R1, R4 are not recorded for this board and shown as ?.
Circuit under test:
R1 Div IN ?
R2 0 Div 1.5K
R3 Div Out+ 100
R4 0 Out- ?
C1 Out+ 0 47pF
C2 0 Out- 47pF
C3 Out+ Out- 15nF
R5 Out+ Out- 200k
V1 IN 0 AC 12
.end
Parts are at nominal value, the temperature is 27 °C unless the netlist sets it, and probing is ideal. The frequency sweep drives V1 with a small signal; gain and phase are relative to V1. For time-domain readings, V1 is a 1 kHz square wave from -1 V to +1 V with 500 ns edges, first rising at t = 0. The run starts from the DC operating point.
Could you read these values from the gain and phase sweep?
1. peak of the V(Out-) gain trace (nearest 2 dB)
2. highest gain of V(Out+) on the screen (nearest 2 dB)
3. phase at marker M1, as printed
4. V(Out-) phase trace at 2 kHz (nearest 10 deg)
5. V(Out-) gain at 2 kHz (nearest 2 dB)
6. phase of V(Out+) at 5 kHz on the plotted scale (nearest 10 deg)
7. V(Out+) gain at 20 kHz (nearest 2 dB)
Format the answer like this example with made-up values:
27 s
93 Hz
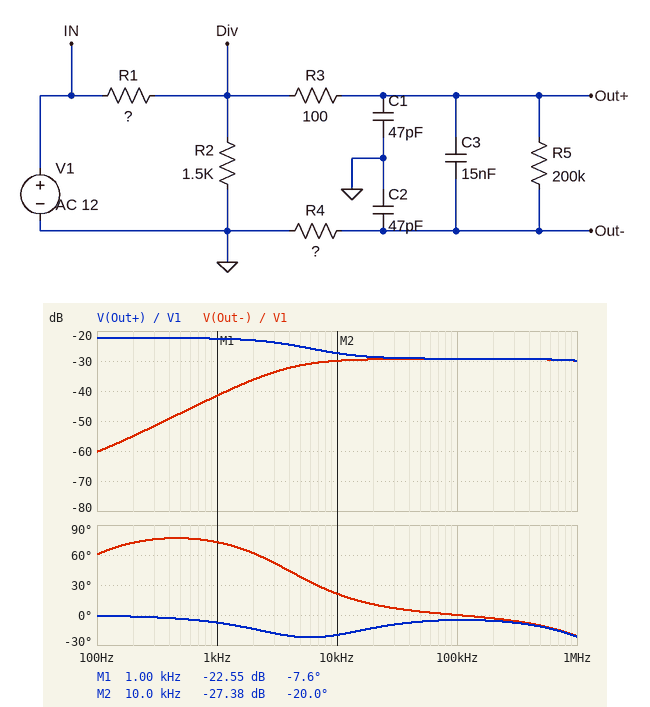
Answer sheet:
-30 dB
-22 dB
-7.6 deg
60 deg
-36 dB
-20 deg
-28 dB
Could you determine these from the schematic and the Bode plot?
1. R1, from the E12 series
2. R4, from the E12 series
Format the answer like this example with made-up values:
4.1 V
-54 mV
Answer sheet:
18 kΩ
1.2 kΩ
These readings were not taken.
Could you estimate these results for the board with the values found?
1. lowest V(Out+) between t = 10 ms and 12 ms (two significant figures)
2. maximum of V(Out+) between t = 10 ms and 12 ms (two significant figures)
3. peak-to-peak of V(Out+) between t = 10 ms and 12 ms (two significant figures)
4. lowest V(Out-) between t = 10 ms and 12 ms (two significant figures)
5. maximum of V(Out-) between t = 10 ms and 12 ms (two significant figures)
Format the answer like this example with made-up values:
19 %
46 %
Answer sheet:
-76 mV
76 mV
150 mV
-67 mV
67 mV
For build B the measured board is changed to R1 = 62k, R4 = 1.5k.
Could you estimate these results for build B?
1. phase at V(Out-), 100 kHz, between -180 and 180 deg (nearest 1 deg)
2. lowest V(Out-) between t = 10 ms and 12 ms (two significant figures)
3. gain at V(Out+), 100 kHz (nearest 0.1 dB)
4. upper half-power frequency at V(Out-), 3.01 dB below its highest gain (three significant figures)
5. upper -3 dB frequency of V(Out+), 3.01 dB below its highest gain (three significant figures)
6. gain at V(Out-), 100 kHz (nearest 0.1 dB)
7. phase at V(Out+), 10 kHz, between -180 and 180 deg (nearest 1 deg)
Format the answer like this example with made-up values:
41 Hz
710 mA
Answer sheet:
-1 deg
-23 mV
-38.7 dB
2.22 MHz
4.91 kHz
-38.8 dB
-16 deg
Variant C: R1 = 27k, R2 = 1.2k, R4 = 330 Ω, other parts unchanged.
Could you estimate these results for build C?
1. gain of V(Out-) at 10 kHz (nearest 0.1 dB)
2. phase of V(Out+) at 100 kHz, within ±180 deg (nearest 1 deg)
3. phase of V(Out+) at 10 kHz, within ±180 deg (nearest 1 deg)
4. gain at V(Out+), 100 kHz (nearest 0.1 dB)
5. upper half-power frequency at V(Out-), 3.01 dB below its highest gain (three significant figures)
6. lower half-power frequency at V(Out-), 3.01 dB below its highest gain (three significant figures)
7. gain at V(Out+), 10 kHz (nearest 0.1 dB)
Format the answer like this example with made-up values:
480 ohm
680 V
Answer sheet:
-42.7 dB
-15 deg
-39 deg
-40.6 dB
6.50 MHz
6.74 kHz
-32.1 dB
